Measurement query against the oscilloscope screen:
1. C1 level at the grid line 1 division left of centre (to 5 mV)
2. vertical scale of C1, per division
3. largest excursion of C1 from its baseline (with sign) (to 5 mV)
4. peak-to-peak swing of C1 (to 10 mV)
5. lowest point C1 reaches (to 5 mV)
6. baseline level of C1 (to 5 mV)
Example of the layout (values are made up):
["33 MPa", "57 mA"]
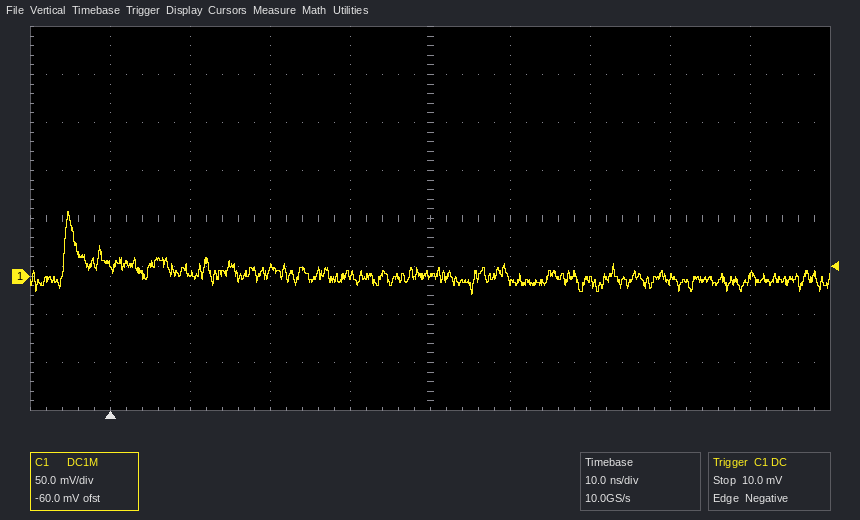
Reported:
["0 mV", "50 mV", "+70 mV", "90 mV", "-20 mV", "0 mV"]
